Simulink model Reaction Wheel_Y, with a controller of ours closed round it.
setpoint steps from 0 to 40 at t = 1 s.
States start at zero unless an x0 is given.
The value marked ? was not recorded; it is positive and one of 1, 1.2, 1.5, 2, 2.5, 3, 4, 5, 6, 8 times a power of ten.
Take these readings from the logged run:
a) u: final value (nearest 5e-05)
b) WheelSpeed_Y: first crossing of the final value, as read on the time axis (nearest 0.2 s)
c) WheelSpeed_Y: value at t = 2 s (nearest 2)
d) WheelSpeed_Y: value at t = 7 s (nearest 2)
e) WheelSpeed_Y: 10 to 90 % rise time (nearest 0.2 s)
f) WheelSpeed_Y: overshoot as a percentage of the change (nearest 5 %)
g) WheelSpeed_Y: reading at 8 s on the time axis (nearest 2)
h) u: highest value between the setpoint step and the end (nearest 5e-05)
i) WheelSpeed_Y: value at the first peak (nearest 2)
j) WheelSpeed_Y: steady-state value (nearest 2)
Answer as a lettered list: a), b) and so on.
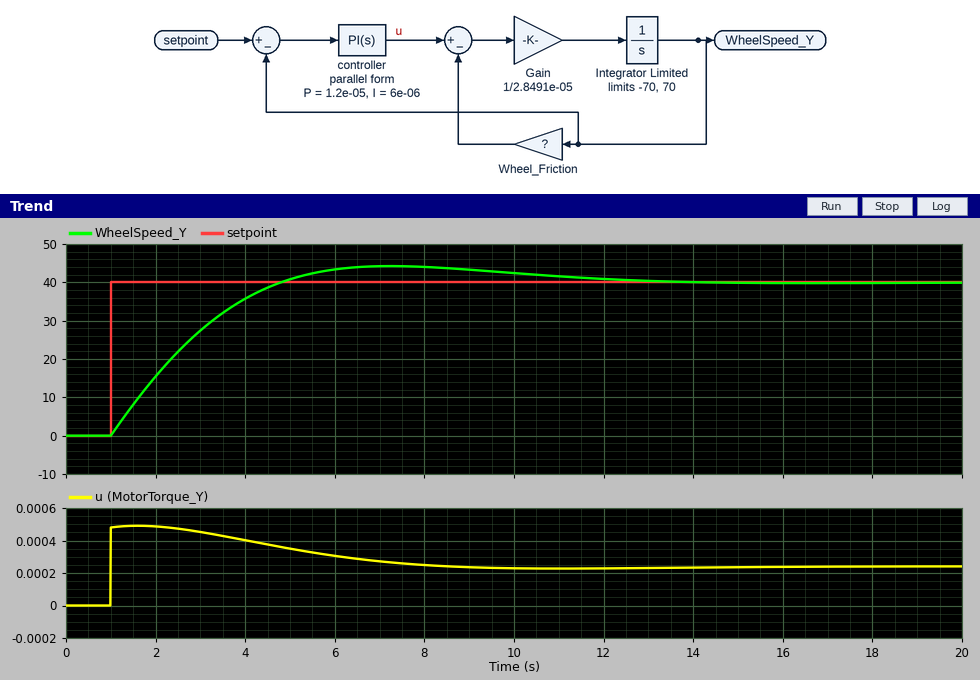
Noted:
a) 0.00025
b) 4.8 s
c) 16
d) 44
e) 2.8 s
f) 10 %
g) 44
h) 0.00050
i) 44
j) 40
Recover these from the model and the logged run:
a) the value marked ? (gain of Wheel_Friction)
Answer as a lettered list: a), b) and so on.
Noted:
a) 6e-06
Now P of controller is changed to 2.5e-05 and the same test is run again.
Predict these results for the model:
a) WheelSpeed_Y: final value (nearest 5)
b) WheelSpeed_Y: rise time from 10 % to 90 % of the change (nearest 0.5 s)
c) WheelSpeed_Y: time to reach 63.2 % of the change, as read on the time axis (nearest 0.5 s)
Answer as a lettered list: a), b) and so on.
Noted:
a) 40
b) 2.5 s
c) 2.0 s
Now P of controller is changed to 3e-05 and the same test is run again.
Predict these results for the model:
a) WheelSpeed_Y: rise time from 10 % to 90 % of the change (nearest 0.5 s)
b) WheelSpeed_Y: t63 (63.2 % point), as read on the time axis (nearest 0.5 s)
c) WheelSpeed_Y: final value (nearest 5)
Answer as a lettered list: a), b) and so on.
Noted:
a) 2.0 s
b) 2.0 s
c) 40
